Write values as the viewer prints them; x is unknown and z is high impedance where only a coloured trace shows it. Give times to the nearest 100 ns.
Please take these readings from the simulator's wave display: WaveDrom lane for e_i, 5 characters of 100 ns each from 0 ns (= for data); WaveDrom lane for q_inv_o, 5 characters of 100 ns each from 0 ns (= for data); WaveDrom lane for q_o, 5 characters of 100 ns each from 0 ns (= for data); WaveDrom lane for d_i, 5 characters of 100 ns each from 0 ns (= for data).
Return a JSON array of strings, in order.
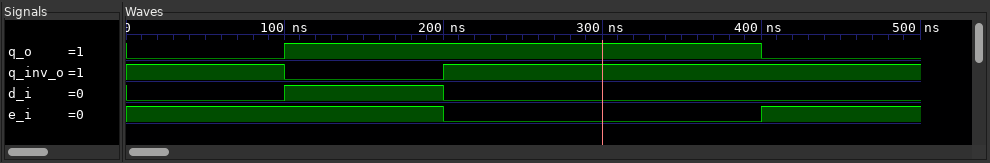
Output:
["{name: 'e_i', wave: '1.0.1'}", "{name: 'q_inv_o', wave: '101..'}", "{name: 'q_o', wave: '01..0'}", "{name: 'd_i', wave: '010..'}"]
